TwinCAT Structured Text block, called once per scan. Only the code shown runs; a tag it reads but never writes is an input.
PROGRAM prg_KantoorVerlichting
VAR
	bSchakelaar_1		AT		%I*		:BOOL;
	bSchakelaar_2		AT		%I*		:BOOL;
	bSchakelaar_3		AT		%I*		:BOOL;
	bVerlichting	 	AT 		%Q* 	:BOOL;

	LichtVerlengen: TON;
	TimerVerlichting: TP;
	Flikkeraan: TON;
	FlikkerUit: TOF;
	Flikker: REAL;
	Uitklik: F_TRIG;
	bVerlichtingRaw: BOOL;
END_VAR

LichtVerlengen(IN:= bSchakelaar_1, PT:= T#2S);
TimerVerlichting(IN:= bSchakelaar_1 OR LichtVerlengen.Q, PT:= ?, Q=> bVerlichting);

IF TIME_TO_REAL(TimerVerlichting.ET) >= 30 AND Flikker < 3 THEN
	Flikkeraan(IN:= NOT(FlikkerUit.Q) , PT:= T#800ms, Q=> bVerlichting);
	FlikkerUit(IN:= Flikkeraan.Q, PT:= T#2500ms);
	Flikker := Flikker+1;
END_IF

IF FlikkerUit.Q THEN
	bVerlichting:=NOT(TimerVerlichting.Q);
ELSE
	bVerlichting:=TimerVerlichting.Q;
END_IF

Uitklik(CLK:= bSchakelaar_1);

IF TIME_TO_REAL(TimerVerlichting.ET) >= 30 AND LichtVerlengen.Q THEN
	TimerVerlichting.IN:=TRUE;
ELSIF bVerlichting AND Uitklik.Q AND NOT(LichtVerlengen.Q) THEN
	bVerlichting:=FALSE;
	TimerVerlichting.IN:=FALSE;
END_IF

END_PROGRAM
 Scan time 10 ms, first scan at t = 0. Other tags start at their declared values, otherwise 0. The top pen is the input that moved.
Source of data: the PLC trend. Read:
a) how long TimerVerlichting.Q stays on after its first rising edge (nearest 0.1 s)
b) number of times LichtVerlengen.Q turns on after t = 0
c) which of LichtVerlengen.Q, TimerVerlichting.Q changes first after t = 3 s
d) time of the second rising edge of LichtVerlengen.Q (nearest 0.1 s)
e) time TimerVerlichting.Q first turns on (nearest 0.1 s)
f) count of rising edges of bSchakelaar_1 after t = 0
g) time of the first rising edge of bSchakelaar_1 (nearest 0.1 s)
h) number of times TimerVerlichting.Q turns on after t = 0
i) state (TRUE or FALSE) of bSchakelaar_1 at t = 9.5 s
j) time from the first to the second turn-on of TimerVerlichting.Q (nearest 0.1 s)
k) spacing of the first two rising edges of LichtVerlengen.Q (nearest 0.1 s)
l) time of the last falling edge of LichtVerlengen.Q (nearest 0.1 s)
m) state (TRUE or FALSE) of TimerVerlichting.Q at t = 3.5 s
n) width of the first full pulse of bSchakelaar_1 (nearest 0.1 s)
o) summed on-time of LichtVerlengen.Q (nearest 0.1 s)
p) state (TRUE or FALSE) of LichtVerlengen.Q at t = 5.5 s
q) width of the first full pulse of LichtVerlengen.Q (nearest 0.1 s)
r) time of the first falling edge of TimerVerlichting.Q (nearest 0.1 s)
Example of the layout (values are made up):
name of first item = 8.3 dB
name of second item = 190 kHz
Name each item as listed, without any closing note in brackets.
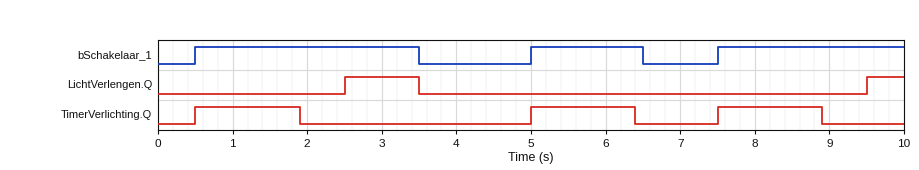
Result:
how long TimerVerlichting.Q stays on after its first rising edge = 1.4 s
number of times LichtVerlengen.Q turns on after t = 0 = 2
which of LichtVerlengen.Q, TimerVerlichting.Q changes first after t = 3 s = LichtVerlengen.Q
time of the second rising edge of LichtVerlengen.Q = 9.5 s
time TimerVerlichting.Q first turns on = 0.5 s
count of rising edges of bSchakelaar_1 after t = 0 = 3
time of the first rising edge of bSchakelaar_1 = 0.5 s
number of times TimerVerlichting.Q turns on after t = 0 = 3
state (TRUE or FALSE) of bSchakelaar_1 at t = 9.5 s = TRUE
time from the first to the second turn-on of TimerVerlichting.Q = 4.5 s
spacing of the first two rising edges of LichtVerlengen.Q = 7.0 s
time of the last falling edge of LichtVerlengen.Q = 3.5 s
state (TRUE or FALSE) of TimerVerlichting.Q at t = 3.5 s = FALSE
width of the first full pulse of bSchakelaar_1 = 3.0 s
summed on-time of LichtVerlengen.Q = 1.5 s
state (TRUE or FALSE) of LichtVerlengen.Q at t = 5.5 s = FALSE
width of the first full pulse of LichtVerlengen.Q = 1.0 s
time of the first falling edge of TimerVerlichting.Q = 1.9 s
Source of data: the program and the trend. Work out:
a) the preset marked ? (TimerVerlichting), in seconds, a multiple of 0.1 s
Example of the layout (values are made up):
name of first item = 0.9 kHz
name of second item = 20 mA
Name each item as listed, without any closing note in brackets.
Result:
the preset marked ? (TimerVerlichting), in seconds, a multiple of 0.1 s = 1.4 s
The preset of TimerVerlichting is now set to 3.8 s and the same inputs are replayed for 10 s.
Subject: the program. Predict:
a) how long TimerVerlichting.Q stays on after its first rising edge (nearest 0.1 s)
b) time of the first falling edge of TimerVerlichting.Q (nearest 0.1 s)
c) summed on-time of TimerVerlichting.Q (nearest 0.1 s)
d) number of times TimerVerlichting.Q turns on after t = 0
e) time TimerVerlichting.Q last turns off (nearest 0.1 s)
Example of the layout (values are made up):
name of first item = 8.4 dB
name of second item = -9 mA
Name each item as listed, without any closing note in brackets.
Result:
how long TimerVerlichting.Q stays on after its first rising edge = 3.8 s
time of the first falling edge of TimerVerlichting.Q = 4.3 s
summed on-time of TimerVerlichting.Q = 7.6 s
number of times TimerVerlichting.Q turns on after t = 0 = 2
time TimerVerlichting.Q last turns off = 8.8 s
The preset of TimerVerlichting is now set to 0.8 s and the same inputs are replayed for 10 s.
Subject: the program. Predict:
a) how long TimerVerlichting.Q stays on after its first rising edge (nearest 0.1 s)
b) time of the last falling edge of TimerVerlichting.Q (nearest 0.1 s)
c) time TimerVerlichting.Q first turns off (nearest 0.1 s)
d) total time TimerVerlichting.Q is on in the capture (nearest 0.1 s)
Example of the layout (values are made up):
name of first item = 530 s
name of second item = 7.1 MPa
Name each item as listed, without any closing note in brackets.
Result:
how long TimerVerlichting.Q stays on after its first rising edge = 0.8 s
time of the last falling edge of TimerVerlichting.Q = 8.3 s
time TimerVerlichting.Q first turns off = 1.3 s
total time TimerVerlichting.Q is on in the capture = 2.4 s
